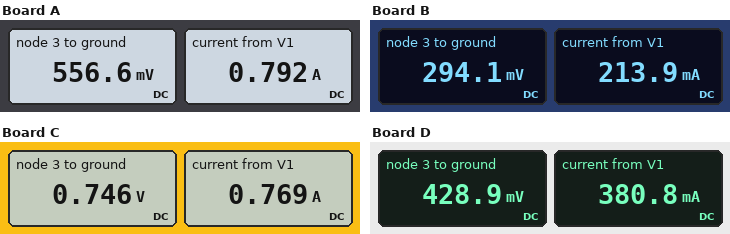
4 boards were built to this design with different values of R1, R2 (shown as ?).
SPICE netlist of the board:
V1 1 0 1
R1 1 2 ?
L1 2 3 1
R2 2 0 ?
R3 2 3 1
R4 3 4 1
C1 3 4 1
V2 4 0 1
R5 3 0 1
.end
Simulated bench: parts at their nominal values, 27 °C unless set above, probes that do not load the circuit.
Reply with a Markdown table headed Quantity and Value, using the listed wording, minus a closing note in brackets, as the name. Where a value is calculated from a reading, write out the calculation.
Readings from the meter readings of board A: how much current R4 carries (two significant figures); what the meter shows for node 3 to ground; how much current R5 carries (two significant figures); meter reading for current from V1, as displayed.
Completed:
| Quantity | Value |
|---|---|
| how much current R4 carries | (1 V - 556.6 mV) / 1 Ω = 440 mA |
| what the meter shows for node 3 to ground | 556.6 mV |
| how much current R5 carries | (556.6 mV) / 1 Ω = 560 mA |
| meter reading for current from V1, as displayed | 0.792 A |
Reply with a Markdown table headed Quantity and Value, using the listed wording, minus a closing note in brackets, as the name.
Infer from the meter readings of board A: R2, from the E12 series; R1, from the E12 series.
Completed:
| Quantity | Value |
|---|---|
| R2, from the E12 series | 0.82 Ω |
| R1, from the E12 series | 0.56 Ω |
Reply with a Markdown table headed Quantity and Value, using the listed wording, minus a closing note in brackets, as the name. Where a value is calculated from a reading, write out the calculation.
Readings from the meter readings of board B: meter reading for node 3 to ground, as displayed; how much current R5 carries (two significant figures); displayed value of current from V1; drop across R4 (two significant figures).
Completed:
| Quantity | Value |
|---|---|
| meter reading for node 3 to ground, as displayed | 294.1 mV |
| how much current R5 carries | (294.1 mV) / 1 Ω = 290 mA |
| displayed value of current from V1 | 213.9 mA |
| drop across R4 | 1 V - 294.1 mV = 710 mV |
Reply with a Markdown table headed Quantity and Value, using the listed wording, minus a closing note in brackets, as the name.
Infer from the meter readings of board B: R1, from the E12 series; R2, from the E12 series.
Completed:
| Quantity | Value |
|---|---|
| R1, from the E12 series | 3.3 Ω |
| R2, from the E12 series | 0.47 Ω |
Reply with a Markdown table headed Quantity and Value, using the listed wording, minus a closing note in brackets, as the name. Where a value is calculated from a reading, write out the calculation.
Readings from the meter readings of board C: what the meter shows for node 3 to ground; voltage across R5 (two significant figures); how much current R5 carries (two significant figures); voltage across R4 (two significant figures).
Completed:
| Quantity | Value |
|---|---|
| what the meter shows for node 3 to ground | 0.746 V |
| voltage across R5 | 746 mV = 750 mV |
| how much current R5 carries | (746 mV) / 1 Ω = 750 mA |
| voltage across R4 | 1 V - 746 mV = 250 mV |
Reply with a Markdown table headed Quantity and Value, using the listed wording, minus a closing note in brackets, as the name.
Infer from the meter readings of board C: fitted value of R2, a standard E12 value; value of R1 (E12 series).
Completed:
| Quantity | Value |
|---|---|
| fitted value of R2, a standard E12 value | 2.7 Ω |
| value of R1 | 0.33 Ω |
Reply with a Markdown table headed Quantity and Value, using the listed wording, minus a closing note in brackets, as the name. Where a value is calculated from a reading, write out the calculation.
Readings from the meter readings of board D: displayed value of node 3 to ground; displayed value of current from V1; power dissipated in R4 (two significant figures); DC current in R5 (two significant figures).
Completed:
| Quantity | Value |
|---|---|
| displayed value of node 3 to ground | 428.9 mV |
| displayed value of current from V1 | 380.8 mA |
| power dissipated in R4 | (1 V - 428.9 mV)^2 / 1 Ω = 330 mW |
| DC current in R5 | (428.9 mV) / 1 Ω = 430 mA |
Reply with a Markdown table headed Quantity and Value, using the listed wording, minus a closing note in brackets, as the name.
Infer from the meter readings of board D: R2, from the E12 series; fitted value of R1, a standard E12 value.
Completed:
| Quantity | Value |
|---|---|
| R2, from the E12 series | 0.82 Ω |
| fitted value of R1, a standard E12 value | 1.5 Ω |
